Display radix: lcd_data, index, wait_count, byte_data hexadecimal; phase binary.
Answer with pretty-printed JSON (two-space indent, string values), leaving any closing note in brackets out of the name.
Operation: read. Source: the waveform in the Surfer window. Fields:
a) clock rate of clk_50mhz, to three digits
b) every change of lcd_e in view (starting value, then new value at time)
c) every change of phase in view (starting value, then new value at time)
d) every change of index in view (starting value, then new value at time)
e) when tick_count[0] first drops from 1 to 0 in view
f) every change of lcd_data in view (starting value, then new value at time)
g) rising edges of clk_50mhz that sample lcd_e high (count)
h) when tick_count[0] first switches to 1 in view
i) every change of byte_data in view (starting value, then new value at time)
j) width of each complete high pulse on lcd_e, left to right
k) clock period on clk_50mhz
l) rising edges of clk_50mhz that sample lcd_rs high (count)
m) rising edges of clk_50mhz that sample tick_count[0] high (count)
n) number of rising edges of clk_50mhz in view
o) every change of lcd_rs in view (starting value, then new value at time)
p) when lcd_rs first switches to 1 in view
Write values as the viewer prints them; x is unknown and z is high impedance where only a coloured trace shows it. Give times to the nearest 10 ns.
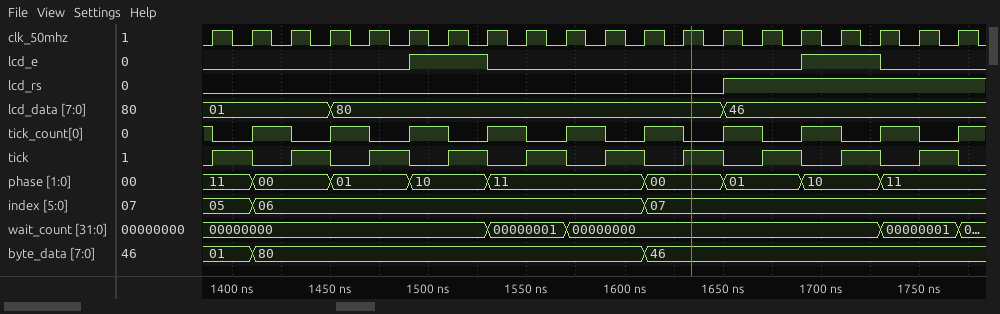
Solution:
{
  "clock rate of clk_50mhz, to three digits": "50.0 MHz",
  "every change of lcd_e in view": "0, 1 at 1490 ns, 0 at 1530 ns, 1 at 1690 ns, 0 at 1730 ns",
  "every change of phase in view": "11, 00 at 1410 ns, 01 at 1450 ns, 10 at 1490 ns, 11 at 1530 ns, 00 at 1610 ns, 01 at 1650 ns, 10 at 1690 ns, 11 at 1730 ns",
  "every change of index in view": "05, 06 at 1410 ns, 07 at 1610 ns",
  "when tick_count[0] first drops from 1 to 0 in view": "1390 ns",
  "every change of lcd_data in view": "01, 80 at 1450 ns, 46 at 1650 ns",
  "rising edges of clk_50mhz that sample lcd_e high": "4",
  "when tick_count[0] first switches to 1 in view": "1410 ns",
  "every change of byte_data in view": "01, 80 at 1410 ns, 46 at 1610 ns",
  "width of each complete high pulse on lcd_e, left to right": "40 ns, 40 ns",
  "clock period on clk_50mhz": "20 ns",
  "rising edges of clk_50mhz that sample lcd_rs high": "6",
  "rising edges of clk_50mhz that sample tick_count[0] high": "10",
  "number of rising edges of clk_50mhz in view": "20",
  "every change of lcd_rs in view": "0, 1 at 1650 ns",
  "when lcd_rs first switches to 1 in view": "1650 ns"
}
